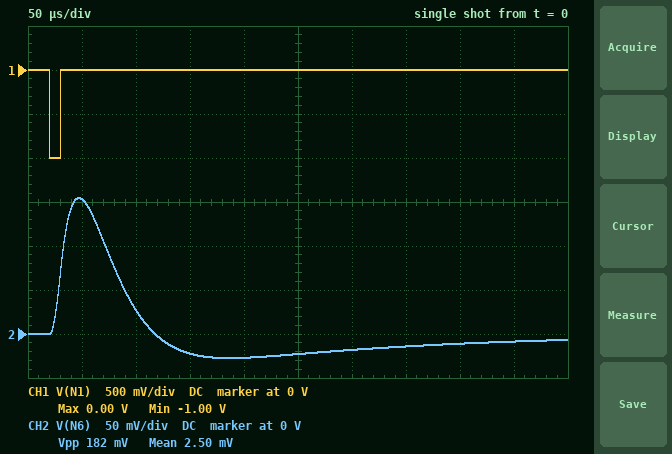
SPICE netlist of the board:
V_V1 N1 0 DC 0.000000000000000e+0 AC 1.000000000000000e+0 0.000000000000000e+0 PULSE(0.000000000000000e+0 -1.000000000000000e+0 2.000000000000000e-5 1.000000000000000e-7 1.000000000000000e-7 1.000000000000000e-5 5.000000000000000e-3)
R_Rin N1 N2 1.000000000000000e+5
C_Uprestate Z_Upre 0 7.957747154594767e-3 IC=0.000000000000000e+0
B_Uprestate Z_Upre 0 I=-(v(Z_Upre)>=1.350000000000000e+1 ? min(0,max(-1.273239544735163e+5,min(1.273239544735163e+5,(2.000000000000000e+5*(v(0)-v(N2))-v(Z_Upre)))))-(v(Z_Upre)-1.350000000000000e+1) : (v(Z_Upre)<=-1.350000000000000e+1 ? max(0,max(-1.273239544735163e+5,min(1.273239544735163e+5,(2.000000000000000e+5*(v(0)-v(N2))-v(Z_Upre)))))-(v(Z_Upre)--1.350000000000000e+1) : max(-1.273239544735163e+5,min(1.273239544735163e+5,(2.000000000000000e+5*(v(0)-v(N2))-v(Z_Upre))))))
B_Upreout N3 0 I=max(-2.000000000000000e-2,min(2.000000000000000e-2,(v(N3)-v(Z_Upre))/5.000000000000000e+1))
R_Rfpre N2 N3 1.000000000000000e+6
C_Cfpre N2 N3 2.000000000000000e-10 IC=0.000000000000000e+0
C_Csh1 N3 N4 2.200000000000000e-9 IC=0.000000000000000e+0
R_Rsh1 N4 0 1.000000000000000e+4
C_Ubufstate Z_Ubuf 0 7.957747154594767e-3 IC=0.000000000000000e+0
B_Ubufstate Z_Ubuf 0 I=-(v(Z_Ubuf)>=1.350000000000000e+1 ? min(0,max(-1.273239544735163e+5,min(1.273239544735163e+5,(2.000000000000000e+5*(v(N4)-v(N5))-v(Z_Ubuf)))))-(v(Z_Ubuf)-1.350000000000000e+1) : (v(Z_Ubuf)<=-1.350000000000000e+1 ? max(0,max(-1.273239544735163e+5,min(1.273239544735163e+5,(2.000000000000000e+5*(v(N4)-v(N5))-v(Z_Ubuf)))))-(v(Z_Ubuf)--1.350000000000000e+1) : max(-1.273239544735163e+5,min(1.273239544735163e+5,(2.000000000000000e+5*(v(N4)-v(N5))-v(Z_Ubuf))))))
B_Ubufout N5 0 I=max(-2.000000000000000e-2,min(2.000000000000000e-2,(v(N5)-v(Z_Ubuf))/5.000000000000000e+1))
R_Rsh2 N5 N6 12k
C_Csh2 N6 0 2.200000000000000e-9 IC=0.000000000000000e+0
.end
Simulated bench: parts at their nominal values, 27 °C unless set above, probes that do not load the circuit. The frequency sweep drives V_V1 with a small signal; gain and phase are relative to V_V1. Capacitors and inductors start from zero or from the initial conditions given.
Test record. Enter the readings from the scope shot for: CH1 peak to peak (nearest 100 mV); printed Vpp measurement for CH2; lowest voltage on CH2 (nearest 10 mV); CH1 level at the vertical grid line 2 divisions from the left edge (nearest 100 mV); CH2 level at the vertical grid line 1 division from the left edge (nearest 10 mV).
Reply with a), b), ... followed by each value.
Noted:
a) 1.0 V
b) 182 mV
c) -30 mV
d) 0 V
e) 150 mV
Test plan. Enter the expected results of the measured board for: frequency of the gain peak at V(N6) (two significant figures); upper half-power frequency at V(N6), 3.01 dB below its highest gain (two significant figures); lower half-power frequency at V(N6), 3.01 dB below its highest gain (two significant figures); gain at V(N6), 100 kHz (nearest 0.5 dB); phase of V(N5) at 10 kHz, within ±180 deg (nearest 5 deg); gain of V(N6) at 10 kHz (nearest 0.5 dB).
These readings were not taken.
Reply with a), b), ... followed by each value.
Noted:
a) 1.9 kHz
b) 5.3 kHz
c) 610 Hz
d) -46.5 dB
e) 130 deg
f) -9.5 dB
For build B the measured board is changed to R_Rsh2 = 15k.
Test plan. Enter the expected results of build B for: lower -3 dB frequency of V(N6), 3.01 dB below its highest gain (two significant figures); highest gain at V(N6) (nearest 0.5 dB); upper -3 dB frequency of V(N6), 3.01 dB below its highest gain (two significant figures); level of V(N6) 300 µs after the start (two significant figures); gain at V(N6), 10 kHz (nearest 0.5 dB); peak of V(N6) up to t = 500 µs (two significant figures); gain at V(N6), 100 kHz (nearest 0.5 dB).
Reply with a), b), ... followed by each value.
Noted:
a) 590 Hz
b) -1.0 dB
c) 4.7 kHz
d) -19 mV
e) -11.0 dB
f) 140 mV
g) -48.5 dB
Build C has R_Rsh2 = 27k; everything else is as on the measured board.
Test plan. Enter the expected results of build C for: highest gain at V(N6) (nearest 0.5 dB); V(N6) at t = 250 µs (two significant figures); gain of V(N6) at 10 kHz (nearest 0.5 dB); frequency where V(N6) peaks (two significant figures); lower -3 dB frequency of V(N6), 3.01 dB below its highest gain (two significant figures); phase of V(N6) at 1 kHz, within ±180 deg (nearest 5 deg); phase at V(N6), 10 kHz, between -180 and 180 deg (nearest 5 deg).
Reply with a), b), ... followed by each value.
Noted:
a) -1.5 dB
b) -19 mV
c) -15.5 dB
d) 1.4 kHz
e) 520 Hz
f) -170 deg
g) 55 deg
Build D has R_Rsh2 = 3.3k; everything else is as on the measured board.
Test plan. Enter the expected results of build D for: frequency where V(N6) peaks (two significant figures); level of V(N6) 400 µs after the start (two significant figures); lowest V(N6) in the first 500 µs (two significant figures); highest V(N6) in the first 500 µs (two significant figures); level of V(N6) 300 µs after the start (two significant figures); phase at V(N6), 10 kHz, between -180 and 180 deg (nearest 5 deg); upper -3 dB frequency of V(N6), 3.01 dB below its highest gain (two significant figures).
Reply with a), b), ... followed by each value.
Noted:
a) 2.3 kHz
b) -9.9 mV
c) -32 mV
d) 270 mV
e) -16 mV
f) 105 deg
g) 7.9 kHz
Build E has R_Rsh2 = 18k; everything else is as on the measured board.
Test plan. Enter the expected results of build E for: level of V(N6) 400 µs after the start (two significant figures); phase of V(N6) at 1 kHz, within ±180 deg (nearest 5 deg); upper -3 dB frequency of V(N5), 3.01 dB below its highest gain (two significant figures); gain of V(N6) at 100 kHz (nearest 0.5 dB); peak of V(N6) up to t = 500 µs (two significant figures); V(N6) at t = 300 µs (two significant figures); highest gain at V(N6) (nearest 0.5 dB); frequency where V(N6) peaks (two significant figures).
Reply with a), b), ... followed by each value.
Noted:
a) -12 mV
b) -165 deg
c) 8.7 kHz
d) -50.0 dB
e) 120 mV
f) -19 mV
g) -1.0 dB
h) 1.6 kHz
